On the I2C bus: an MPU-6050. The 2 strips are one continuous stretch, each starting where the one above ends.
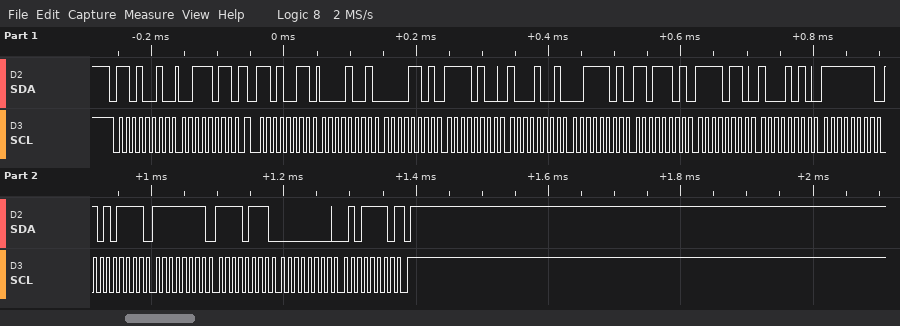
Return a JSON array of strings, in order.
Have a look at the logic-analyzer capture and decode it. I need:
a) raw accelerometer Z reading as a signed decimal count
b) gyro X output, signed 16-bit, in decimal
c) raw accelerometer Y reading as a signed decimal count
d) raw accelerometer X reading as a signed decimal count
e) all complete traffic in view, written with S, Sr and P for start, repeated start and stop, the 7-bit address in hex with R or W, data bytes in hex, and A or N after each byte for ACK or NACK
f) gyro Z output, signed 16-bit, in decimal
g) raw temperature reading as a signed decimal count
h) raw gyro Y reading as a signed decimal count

["15837", "-81", "-2935", "2317", "S 69W A 3B A Sr 69R A 09 A 0D A F4 A 89 A 3D A DD A F6 A 8A A FF A AF A FF A F7 A 00 A 5E N P", "94", "-2422", "-9"]
